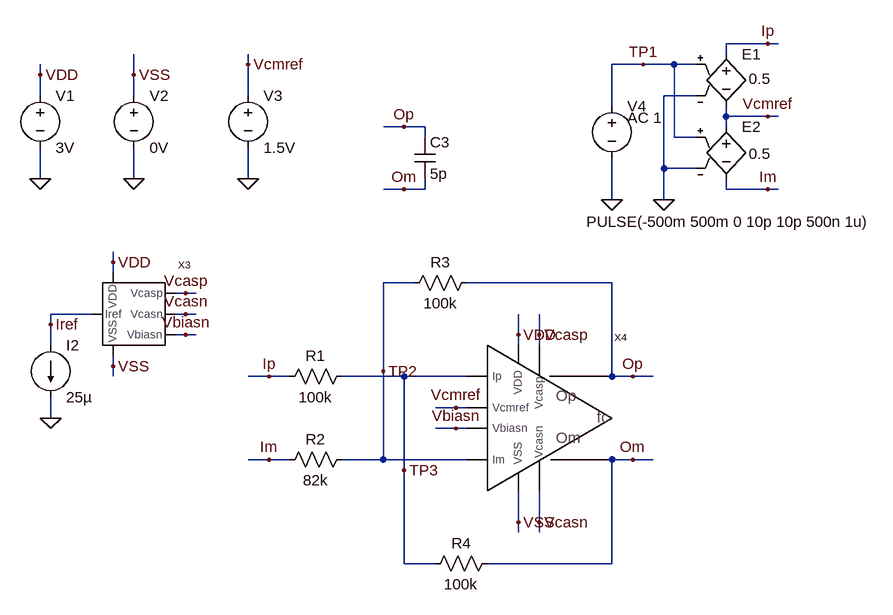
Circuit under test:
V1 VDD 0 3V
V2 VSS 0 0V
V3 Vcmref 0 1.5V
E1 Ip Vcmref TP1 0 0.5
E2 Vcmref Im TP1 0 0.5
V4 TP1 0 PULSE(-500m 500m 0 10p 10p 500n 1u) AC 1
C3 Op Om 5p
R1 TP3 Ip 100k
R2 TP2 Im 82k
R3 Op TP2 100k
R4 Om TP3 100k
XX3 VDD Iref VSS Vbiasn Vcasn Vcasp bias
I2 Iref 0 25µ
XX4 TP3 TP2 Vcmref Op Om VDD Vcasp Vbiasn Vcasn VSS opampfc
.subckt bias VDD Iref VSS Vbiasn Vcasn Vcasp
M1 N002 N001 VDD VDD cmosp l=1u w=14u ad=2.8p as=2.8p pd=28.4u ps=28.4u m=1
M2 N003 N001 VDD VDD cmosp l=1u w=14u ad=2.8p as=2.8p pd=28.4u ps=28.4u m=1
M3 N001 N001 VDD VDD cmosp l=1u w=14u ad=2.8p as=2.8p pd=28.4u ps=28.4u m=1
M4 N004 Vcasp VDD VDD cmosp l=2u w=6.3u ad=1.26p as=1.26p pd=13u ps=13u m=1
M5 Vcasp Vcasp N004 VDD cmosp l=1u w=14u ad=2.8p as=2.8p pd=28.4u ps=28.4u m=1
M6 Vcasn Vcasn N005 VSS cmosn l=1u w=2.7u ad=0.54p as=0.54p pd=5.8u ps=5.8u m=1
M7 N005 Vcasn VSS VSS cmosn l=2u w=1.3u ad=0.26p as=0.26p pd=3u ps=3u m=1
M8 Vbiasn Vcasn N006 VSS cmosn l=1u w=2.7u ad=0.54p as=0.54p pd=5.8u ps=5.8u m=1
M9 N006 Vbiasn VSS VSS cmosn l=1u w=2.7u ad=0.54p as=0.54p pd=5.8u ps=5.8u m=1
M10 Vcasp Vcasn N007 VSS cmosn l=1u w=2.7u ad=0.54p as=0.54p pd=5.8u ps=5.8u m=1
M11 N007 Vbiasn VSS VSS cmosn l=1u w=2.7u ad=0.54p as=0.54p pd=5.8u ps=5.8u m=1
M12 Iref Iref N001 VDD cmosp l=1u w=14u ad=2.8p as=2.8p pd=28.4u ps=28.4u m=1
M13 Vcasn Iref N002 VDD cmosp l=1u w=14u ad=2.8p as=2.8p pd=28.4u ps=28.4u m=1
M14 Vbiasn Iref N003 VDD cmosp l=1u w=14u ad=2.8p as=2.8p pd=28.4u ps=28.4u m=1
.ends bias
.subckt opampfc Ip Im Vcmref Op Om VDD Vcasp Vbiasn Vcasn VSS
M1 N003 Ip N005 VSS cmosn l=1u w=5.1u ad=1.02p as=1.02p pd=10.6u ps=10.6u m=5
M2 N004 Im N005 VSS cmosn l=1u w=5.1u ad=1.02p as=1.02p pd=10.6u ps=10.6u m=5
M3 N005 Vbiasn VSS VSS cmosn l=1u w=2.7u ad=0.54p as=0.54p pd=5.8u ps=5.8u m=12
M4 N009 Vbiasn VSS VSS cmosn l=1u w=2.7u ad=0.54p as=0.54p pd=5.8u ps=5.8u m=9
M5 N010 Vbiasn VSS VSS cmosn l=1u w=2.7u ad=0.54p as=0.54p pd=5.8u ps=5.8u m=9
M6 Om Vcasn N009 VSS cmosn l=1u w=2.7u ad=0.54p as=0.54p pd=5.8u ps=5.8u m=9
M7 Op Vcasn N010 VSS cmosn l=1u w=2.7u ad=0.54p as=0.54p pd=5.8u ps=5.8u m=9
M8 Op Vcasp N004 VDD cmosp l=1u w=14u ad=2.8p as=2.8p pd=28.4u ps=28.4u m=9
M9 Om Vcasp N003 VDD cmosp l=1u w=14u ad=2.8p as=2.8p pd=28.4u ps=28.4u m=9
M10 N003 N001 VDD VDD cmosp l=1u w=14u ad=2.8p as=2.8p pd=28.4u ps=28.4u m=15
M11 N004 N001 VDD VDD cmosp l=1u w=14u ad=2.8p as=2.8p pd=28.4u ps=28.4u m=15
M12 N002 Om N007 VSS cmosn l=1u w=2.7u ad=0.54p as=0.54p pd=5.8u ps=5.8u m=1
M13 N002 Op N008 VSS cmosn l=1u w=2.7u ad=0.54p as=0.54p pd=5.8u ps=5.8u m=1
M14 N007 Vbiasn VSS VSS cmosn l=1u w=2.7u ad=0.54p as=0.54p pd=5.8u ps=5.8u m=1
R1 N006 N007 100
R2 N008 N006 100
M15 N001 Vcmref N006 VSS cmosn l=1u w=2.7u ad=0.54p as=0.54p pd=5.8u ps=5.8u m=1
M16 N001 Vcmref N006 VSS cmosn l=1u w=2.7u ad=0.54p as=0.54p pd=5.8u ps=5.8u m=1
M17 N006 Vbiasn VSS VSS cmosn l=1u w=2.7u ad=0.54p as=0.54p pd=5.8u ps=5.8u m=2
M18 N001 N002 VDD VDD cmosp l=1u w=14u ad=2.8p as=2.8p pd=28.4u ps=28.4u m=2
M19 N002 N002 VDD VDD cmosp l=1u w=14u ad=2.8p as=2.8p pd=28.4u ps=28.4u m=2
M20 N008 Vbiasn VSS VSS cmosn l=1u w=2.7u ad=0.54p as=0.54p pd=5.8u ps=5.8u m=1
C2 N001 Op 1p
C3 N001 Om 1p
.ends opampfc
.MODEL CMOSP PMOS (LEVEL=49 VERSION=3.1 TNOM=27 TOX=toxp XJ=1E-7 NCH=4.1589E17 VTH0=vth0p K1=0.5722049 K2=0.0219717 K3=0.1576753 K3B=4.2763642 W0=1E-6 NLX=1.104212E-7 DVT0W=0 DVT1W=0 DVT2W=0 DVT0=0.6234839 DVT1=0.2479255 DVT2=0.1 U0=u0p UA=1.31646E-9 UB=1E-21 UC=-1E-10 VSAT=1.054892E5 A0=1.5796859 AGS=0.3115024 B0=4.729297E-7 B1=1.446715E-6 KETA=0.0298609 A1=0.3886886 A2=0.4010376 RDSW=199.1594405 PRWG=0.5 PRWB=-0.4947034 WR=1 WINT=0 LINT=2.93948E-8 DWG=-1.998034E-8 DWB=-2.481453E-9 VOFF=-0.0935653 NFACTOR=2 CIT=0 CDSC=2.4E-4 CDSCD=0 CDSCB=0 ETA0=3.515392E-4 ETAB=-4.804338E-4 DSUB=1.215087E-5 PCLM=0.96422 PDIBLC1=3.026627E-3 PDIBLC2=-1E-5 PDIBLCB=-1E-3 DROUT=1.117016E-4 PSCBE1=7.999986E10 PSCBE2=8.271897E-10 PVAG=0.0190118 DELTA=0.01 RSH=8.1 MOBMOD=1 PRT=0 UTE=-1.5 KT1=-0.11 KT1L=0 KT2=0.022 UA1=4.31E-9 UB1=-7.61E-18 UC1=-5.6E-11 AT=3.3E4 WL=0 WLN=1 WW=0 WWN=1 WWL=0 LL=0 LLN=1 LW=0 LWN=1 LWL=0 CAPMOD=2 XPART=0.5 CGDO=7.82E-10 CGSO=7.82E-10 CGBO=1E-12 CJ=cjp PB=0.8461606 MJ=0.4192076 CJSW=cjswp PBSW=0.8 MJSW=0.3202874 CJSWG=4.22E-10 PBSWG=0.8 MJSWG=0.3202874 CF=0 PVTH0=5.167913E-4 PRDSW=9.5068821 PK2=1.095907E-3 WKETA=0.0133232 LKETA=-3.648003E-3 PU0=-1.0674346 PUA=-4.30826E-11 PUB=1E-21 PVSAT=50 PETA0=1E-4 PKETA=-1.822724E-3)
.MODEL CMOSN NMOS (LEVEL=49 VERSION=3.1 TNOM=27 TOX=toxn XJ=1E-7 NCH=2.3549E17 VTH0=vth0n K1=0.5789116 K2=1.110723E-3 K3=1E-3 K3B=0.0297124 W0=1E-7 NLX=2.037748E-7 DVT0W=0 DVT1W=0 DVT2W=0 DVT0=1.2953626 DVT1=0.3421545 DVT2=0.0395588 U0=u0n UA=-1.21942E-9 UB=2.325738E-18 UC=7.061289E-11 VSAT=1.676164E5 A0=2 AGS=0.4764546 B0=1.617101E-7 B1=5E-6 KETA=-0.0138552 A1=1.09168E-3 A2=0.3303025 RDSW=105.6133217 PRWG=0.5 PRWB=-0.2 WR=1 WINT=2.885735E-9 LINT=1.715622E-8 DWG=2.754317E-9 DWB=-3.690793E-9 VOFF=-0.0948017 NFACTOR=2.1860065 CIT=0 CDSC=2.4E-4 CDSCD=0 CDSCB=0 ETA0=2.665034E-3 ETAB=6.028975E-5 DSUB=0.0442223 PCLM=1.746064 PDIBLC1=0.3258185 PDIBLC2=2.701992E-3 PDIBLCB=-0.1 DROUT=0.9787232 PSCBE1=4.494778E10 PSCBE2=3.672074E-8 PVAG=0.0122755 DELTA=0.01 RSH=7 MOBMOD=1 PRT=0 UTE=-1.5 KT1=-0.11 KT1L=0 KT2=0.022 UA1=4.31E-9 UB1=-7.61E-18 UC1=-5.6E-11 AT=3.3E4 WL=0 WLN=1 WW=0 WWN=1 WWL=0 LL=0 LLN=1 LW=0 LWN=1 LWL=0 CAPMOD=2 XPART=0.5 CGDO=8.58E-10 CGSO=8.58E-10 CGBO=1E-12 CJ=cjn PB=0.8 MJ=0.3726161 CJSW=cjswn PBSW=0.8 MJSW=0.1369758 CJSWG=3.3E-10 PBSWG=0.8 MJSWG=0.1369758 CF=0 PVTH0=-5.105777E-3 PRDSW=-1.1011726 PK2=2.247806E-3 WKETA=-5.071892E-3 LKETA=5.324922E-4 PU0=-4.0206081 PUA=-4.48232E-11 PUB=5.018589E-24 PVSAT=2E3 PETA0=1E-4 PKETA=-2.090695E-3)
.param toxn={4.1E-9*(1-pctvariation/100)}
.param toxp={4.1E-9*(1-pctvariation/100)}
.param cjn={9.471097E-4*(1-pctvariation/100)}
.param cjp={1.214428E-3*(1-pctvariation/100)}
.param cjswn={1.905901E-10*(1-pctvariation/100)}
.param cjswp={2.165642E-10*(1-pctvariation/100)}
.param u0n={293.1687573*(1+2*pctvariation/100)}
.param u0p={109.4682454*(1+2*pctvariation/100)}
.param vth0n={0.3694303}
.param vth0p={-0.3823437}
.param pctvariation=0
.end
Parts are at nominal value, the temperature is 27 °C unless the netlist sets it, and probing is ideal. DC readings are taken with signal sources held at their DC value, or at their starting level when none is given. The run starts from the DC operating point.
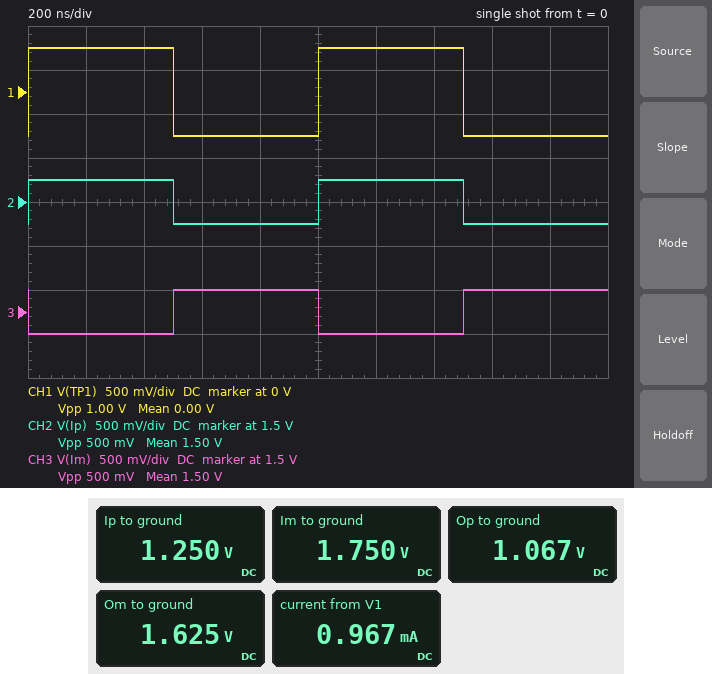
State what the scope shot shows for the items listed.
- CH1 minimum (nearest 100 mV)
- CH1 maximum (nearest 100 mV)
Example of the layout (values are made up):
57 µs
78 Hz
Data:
-500 mV
500 mV
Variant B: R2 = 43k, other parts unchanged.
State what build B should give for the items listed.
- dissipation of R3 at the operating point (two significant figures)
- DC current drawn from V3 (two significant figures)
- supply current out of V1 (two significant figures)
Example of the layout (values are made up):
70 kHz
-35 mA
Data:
5.0 µW
5.2 µA
960 µA
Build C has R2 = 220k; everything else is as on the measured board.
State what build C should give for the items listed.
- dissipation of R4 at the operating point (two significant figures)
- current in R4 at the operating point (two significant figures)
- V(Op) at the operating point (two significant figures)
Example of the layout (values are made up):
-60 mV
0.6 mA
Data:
330 nW
1.8 µA
1.3 V
